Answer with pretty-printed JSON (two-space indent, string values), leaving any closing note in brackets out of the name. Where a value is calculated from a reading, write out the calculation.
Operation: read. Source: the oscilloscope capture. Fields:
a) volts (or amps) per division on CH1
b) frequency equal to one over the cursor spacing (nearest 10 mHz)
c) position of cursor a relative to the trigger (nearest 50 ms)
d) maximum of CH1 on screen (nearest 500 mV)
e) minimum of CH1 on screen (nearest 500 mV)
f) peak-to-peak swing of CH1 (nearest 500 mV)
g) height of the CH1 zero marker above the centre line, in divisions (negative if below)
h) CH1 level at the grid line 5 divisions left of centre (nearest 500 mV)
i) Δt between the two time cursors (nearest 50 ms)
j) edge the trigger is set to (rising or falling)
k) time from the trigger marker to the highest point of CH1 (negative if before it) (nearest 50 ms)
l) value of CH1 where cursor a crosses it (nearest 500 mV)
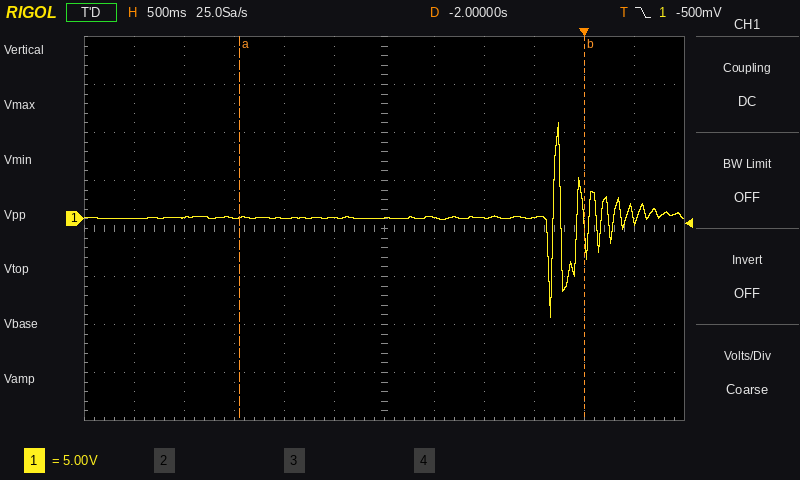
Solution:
{
  "volts (or amps) per division on CH1": "5 V",
  "frequency equal to one over the cursor spacing": "1 / 3.45 s ≈ 290 mHz",
  "position of cursor a relative to the trigger": "-3.45 s",
  "maximum of CH1 on screen": "10.0 V",
  "minimum of CH1 on screen": "-10.5 V",
  "peak-to-peak swing of CH1": "10.0 V − (-10.5 V) = 20.5 V",
  "height of the CH1 zero marker above the centre line, in divisions": "+0.2 div",
  "CH1 level at the grid line 5 divisions left of centre": "0.0 V",
  "Δt between the two time cursors": "3.45 s",
  "edge the trigger is set to": "falling",
  "time from the trigger marker to the highest point of CH1 (negative if before it)": "-250 ms",
  "value of CH1 where cursor a crosses it": "0.0 V"
}
